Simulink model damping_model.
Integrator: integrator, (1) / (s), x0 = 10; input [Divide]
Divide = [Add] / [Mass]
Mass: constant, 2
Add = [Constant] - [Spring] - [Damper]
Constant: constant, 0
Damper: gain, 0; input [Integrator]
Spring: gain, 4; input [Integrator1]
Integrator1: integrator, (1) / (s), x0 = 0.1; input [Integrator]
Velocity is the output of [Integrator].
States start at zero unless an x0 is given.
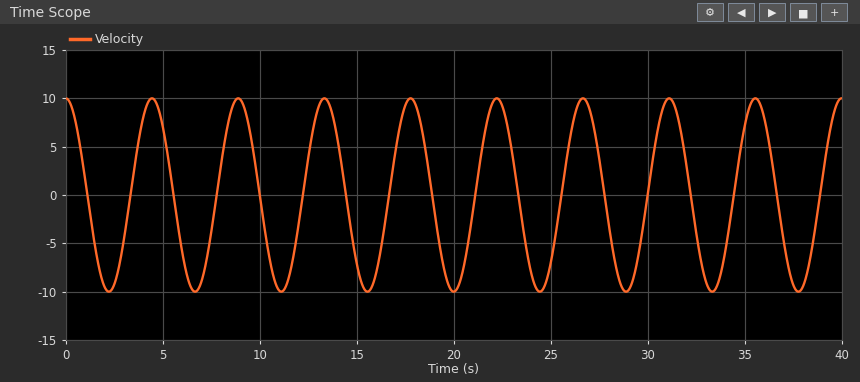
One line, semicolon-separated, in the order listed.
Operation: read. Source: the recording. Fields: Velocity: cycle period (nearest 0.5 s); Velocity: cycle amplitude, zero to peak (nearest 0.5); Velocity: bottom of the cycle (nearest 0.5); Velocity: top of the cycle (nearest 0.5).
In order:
4.5 s; 10.0; -10.0; 10.0
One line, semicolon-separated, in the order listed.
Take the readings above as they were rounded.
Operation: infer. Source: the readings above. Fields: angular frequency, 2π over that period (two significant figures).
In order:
1.4 rad/s
